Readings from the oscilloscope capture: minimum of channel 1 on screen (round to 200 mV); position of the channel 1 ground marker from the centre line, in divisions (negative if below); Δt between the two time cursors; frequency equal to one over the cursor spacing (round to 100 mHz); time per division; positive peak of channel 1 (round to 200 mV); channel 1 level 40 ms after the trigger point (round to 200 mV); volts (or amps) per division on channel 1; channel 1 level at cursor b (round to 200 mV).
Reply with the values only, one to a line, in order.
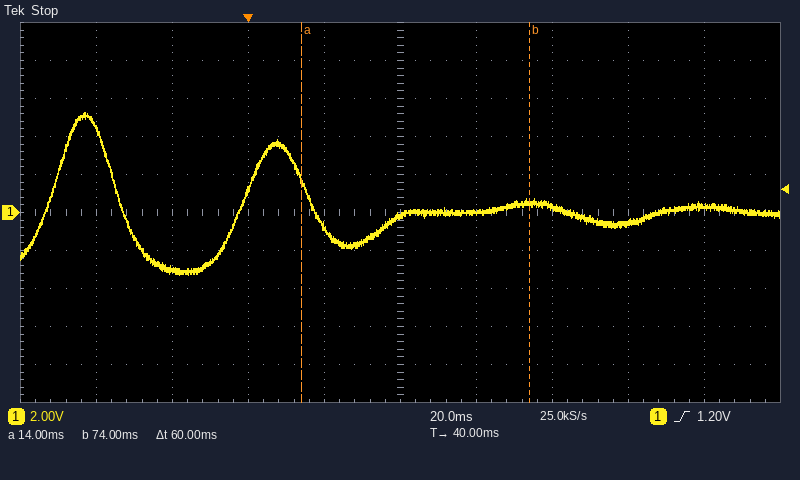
-3.2 V
0.0 div
60 ms
16.7 Hz
20 ms
5.2 V
-200 mV
2 V
600 mV
